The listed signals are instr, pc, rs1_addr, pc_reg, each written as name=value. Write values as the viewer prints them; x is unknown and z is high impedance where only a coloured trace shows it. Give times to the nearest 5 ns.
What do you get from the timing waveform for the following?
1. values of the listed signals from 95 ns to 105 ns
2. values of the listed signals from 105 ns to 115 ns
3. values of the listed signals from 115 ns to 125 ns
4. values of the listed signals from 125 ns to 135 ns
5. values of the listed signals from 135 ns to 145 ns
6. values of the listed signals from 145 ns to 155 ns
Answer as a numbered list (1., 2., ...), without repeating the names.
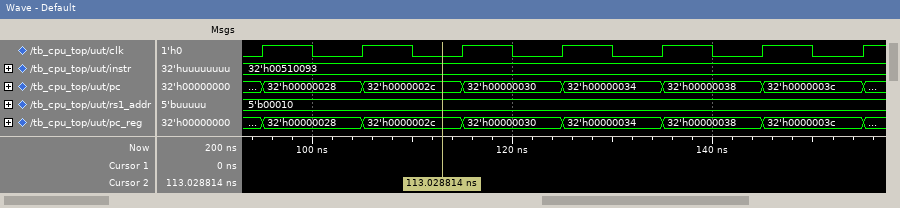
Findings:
1. instr=32'h00510093, pc=32'h00000028, rs1_addr=5'b00010, pc_reg=32'h00000028
2. instr=32'h00510093, pc=32'h0000002c, rs1_addr=5'b00010, pc_reg=32'h0000002c
3. instr=32'h00510093, pc=32'h00000030, rs1_addr=5'b00010, pc_reg=32'h00000030
4. instr=32'h00510093, pc=32'h00000034, rs1_addr=5'b00010, pc_reg=32'h00000034
5. instr=32'h00510093, pc=32'h00000038, rs1_addr=5'b00010, pc_reg=32'h00000038
6. instr=32'h00510093, pc=32'h0000003c, rs1_addr=5'b00010, pc_reg=32'h0000003c
